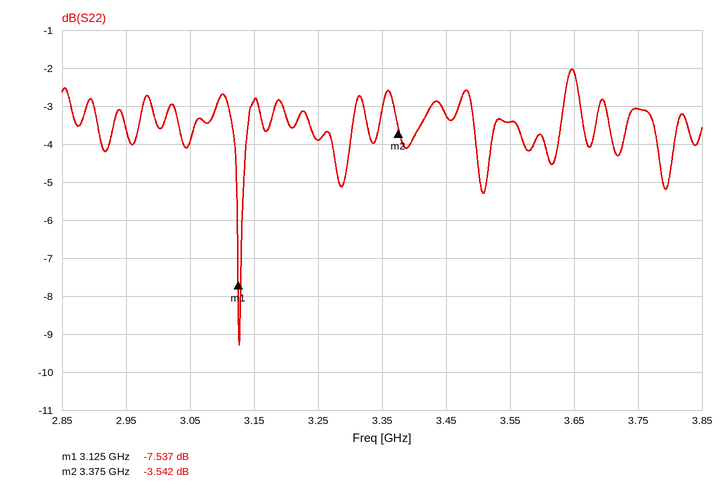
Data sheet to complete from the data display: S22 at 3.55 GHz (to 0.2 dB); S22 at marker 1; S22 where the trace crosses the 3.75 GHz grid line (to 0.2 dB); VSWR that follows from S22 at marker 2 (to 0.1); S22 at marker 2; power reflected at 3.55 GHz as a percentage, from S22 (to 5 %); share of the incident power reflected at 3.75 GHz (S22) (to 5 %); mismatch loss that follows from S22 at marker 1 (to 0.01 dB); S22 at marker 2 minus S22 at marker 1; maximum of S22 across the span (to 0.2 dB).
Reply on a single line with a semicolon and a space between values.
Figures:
-3.4 dB; -7.537 dB; -3.0 dB; 5.0; -3.542 dB; 45 %; 50 %; 0.84 dB; 3.995 dB; -2.0 dB
